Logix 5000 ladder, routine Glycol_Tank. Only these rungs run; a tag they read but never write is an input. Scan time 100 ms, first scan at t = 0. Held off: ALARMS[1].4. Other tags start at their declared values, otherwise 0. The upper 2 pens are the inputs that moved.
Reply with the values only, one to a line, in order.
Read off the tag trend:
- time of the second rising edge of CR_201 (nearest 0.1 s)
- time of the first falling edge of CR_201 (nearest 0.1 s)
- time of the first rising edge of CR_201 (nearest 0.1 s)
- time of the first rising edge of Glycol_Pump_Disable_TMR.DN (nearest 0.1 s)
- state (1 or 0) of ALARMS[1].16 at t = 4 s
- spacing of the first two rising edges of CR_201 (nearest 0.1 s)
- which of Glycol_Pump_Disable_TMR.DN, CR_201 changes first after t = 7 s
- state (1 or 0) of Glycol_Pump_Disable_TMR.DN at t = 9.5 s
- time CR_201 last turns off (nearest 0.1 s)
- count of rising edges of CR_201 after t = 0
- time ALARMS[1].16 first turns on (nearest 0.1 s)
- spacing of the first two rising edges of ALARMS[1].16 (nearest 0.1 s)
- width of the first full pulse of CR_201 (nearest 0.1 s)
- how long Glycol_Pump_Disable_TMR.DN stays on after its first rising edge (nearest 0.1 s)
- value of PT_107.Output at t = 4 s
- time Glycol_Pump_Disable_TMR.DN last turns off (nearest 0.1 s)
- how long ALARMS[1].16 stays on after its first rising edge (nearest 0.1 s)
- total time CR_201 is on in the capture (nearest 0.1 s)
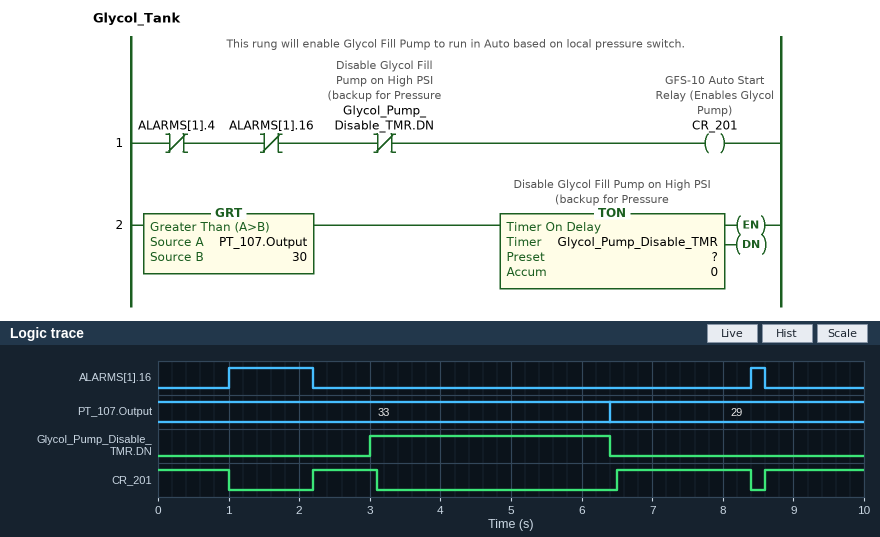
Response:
6.5 s
1.0 s
2.2 s
3.0 s
0
4.3 s
CR_201
0
8.4 s
3
1.0 s
7.4 s
0.9 s
3.4 s
33
6.4 s
1.2 s
5.2 s
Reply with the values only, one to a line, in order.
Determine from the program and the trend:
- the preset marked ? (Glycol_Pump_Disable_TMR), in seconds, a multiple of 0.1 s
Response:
3.0 s
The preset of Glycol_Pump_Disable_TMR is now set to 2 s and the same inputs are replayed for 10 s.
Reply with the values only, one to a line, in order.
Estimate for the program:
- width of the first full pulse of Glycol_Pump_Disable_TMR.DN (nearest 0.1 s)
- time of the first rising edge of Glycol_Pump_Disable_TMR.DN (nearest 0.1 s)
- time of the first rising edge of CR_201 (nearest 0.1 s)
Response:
4.4 s
2.0 s
6.5 s
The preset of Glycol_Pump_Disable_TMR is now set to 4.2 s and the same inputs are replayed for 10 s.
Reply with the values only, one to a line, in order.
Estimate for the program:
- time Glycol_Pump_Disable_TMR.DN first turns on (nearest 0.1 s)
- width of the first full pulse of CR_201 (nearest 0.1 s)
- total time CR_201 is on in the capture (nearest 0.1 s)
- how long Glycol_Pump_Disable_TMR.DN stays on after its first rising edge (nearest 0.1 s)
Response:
4.2 s
2.1 s
6.4 s
2.2 s
